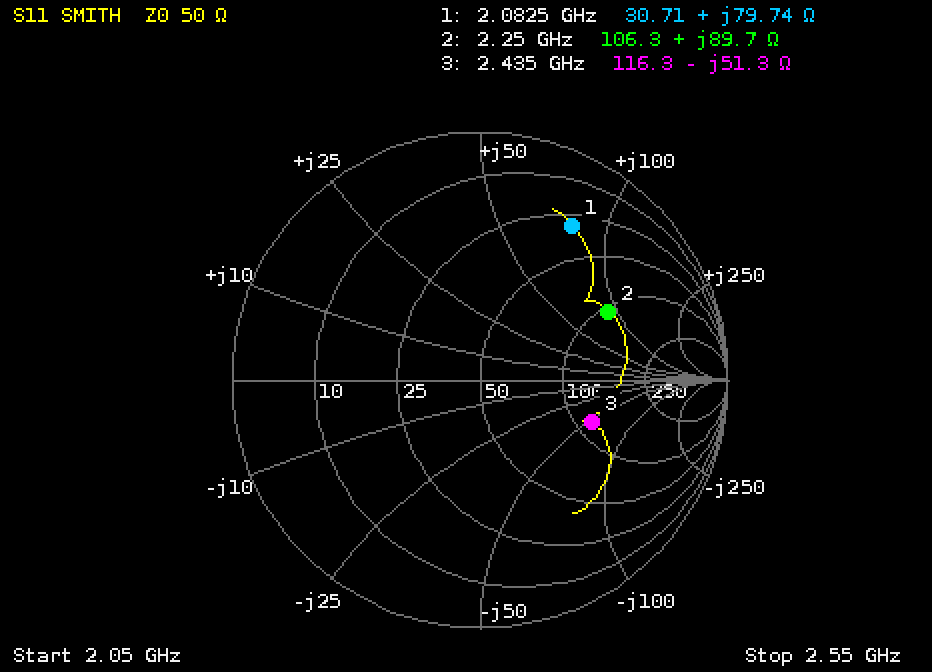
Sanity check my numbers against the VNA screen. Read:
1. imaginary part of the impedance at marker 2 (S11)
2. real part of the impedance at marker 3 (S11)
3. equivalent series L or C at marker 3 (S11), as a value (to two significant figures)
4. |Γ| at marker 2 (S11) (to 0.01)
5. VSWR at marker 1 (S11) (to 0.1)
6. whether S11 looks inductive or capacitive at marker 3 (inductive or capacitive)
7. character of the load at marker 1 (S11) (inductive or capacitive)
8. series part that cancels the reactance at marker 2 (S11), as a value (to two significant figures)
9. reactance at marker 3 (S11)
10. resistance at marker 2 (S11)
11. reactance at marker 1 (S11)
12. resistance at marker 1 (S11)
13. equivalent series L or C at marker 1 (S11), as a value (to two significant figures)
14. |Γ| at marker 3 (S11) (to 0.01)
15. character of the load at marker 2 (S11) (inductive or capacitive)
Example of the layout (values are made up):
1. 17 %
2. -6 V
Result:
1. +89.7 Ω
2. 116.3 Ω
3. 1.3 pF
4. 0.59
5. 6.2
6. capacitive
7. inductive
8. 790 fF
9. -51.3 Ω
10. 106.3 Ω
11. +79.74 Ω
12. 30.71 Ω
13. 6.1 nH
14. 0.48
15. inductive
